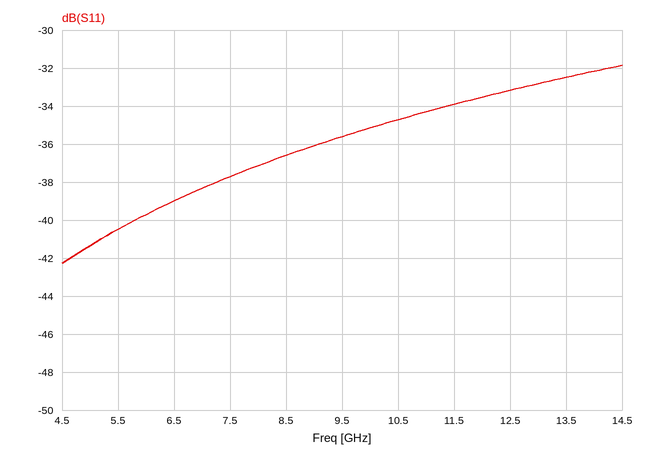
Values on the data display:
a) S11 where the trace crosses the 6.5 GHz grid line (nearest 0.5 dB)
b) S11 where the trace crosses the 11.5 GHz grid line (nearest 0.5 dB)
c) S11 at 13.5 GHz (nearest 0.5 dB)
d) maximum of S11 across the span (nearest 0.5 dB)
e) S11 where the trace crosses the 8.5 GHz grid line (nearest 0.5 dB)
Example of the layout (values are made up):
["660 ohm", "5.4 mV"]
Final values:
["-39.0 dB", "-34.0 dB", "-32.5 dB", "-32.0 dB", "-36.5 dB"]
